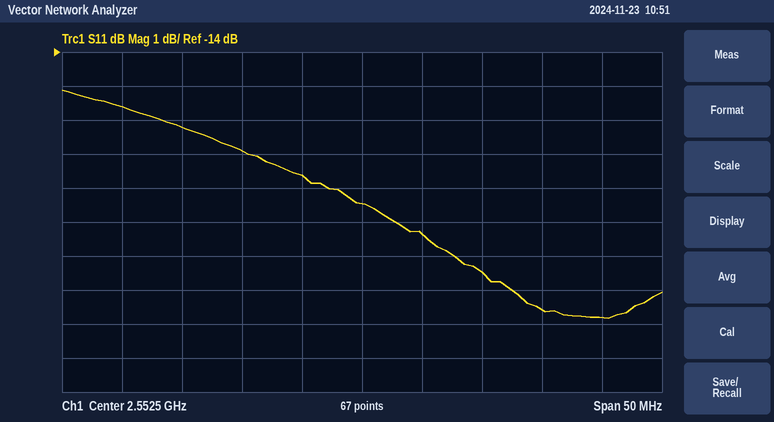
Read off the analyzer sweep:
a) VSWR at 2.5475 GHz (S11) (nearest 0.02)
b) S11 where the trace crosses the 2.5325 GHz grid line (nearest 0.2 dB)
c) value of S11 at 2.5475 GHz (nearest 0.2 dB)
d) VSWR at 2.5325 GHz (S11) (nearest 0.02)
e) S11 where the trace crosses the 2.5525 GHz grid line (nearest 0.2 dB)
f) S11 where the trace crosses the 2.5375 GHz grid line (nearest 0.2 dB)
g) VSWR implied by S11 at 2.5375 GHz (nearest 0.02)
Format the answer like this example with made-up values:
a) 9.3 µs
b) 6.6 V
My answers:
a) 1.30
b) -15.6 dB
c) -17.6 dB
d) 1.40
e) -18.4 dB
f) -16.2 dB
g) 1.36
